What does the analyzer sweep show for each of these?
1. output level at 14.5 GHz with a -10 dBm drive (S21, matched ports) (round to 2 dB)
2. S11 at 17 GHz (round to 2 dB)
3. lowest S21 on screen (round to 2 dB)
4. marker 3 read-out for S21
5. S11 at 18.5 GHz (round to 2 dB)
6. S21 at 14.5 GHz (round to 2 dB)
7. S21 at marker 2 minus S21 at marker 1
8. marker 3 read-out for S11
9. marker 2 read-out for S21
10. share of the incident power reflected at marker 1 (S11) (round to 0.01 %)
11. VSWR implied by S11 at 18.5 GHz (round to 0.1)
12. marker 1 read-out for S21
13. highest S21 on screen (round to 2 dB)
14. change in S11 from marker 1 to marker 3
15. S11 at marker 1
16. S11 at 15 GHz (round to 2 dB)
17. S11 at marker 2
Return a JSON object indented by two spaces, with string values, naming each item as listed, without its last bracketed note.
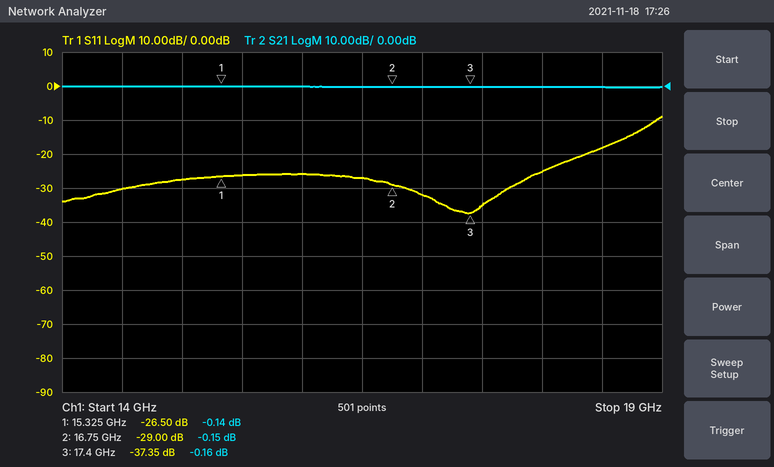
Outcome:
{
  "output level at 14.5 GHz with a -10 dBm drive (S21, matched ports)": "-10 dBm",
  "S11 at 17 GHz": "-32 dB",
  "lowest S21 on screen": "0 dB",
  "marker 3 read-out for S21": "-0.16 dB",
  "S11 at 18.5 GHz": "-18 dB",
  "S21 at 14.5 GHz": "0 dB",
  "S21 at marker 2 minus S21 at marker 1": "-0.01 dB",
  "marker 3 read-out for S11": "-37.35 dB",
  "marker 2 read-out for S21": "-0.15 dB",
  "share of the incident power reflected at marker 1 (S11)": "0.22 %",
  "VSWR implied by S11 at 18.5 GHz": "1.3",
  "marker 1 read-out for S21": "-0.14 dB",
  "highest S21 on screen": "0 dB",
  "change in S11 from marker 1 to marker 3": "-10.85 dB",
  "S11 at marker 1": "-26.50 dB",
  "S11 at 15 GHz": "-28 dB",
  "S11 at marker 2": "-29.00 dB"
}
